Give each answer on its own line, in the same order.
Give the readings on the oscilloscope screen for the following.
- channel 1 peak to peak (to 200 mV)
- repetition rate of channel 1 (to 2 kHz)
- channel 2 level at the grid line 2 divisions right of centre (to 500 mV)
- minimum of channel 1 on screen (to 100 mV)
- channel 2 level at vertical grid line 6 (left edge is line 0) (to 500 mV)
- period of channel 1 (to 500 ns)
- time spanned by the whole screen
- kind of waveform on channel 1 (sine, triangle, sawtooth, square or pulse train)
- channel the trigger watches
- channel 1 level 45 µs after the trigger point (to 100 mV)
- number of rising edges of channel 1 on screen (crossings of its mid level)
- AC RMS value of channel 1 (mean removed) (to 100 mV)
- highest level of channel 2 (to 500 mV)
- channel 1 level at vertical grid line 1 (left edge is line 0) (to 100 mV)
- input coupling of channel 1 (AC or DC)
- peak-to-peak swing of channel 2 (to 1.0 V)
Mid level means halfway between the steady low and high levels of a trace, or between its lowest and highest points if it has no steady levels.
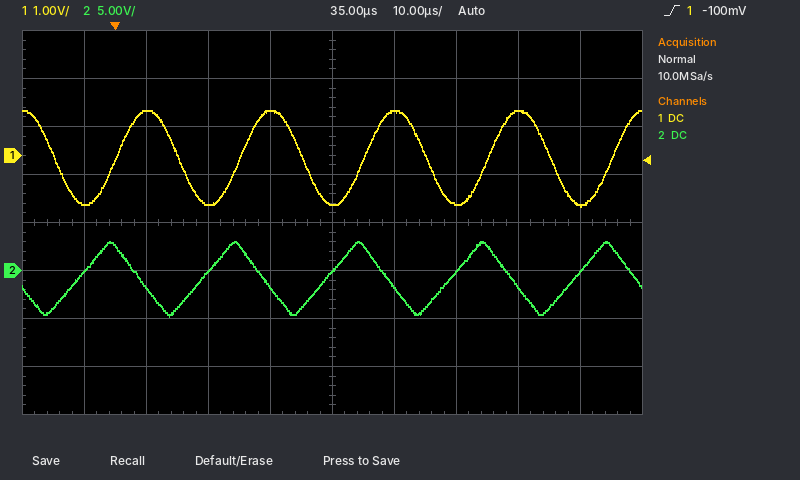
2.0 V
50 kHz
0.0 V
-1.1 V
-1.5 V
20.0 µs
100 µs
sine
channel 1
900 mV
5
700 mV
3.0 V
-1.0 V
DC
8.0 V
